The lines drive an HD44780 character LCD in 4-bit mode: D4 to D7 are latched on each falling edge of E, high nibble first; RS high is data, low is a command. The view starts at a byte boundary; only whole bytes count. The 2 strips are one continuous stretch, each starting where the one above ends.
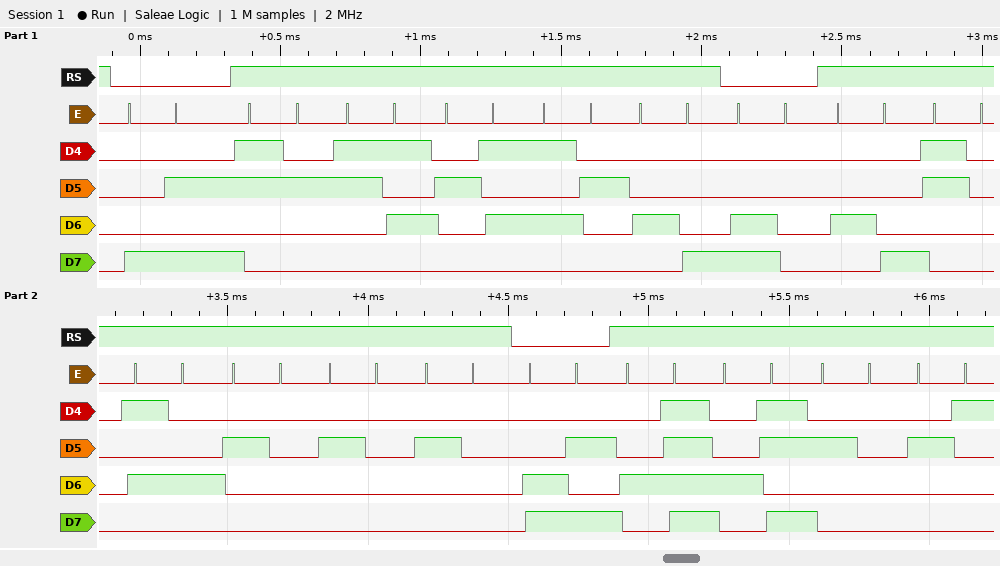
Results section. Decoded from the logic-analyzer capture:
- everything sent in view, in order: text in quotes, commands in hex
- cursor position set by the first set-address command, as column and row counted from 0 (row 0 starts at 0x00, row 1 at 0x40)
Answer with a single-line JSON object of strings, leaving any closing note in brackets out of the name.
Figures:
{"everything sent in view, in order: text in quotes, commands in hex": "0x8A \"25%RH\" 0xC0 \"H0T   \" 0xCA \"OK !\"", "cursor position set by the first set-address command, as column and row counted from 0": "column 10, row 0"}
